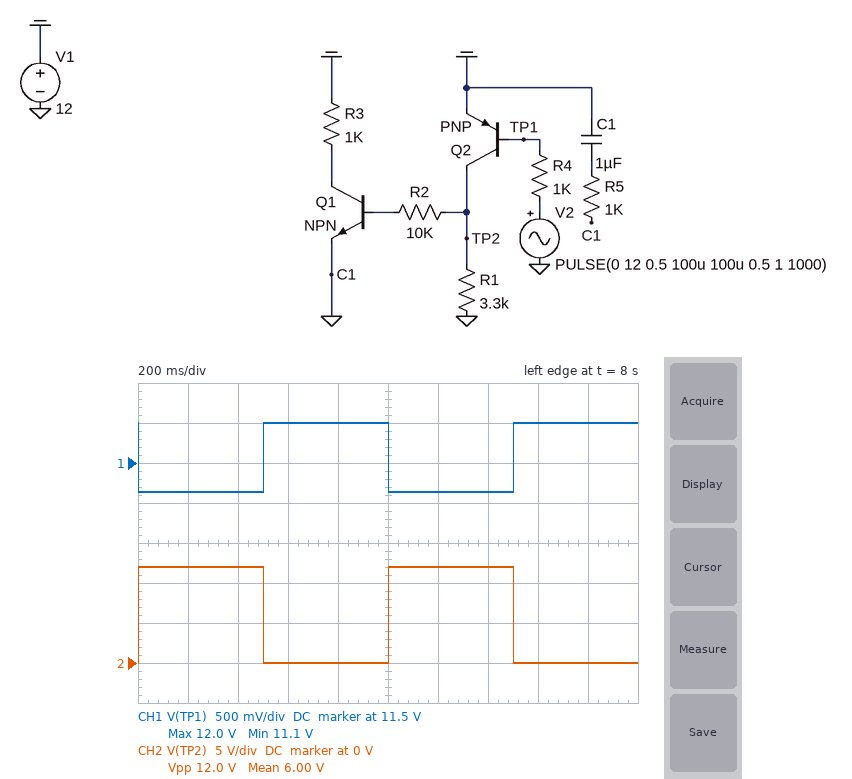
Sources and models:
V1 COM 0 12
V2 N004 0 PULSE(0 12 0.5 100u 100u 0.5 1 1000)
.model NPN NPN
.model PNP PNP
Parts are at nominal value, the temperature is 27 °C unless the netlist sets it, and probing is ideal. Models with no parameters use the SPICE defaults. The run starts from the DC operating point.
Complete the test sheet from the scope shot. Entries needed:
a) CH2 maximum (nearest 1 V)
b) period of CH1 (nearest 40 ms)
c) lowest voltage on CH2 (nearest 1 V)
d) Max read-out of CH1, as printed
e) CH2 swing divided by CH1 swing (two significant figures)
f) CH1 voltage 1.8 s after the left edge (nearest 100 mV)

12 V
1.00 s
0 V
12.0 V
14
12.0 V
